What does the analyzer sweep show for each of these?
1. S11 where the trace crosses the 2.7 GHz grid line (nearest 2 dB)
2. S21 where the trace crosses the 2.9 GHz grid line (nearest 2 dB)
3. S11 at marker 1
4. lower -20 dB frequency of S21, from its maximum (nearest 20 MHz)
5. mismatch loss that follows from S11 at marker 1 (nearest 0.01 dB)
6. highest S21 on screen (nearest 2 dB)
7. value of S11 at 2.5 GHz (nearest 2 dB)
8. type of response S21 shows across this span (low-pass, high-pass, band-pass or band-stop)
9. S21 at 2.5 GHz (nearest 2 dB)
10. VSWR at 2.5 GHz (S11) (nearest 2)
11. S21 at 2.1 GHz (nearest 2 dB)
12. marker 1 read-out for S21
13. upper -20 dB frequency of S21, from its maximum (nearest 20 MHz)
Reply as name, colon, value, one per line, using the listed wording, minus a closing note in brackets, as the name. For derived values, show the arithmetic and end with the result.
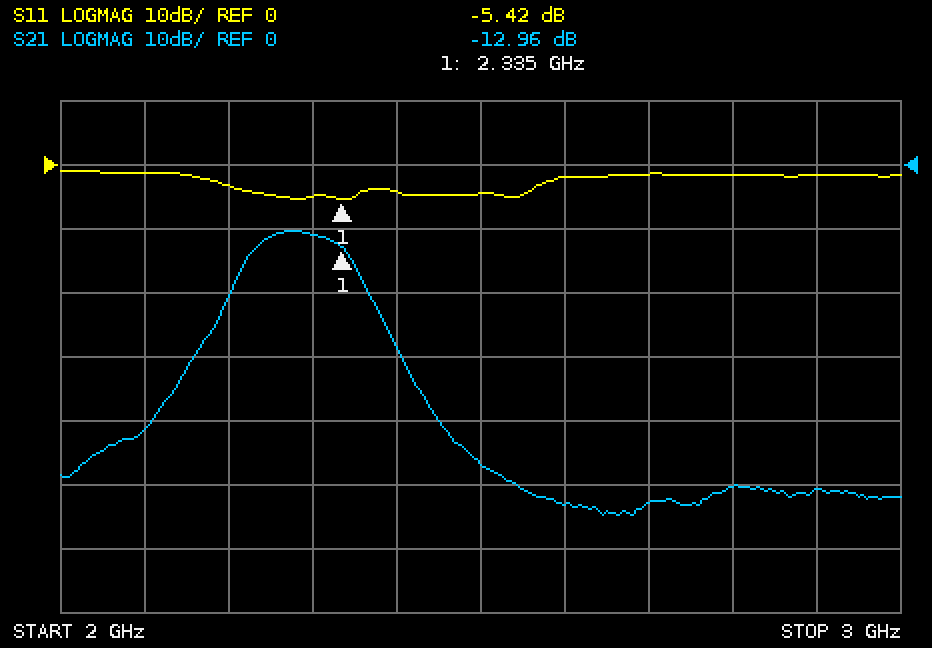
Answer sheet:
S11 where the trace crosses the 2.7 GHz grid line: -2 dB
S21 where the trace crosses the 2.9 GHz grid line: -50 dB
S11 at marker 1: -5.42 dB
lower -20 dB frequency of S21, from its maximum: 2.16 GHz
mismatch loss that follows from S11 at marker 1: −10 log10(1 − 10^(-5.42/10)) ≈ 1.47 dB
highest S21 on screen: -10 dB
value of S11 at 2.5 GHz: -4 dB
type of response S21 shows across this span: band-pass
S21 at 2.5 GHz: -46 dB
VSWR at 2.5 GHz (S11): |Γ| = 10^(-4/20) = 0.6310; VSWR = (1 + 0.6310)/(1 − 0.6310) ≈ 4
S21 at 2.1 GHz: -42 dB
marker 1 read-out for S21: -12.96 dB
upper -20 dB frequency of S21, from its maximum: 2.40 GHz
